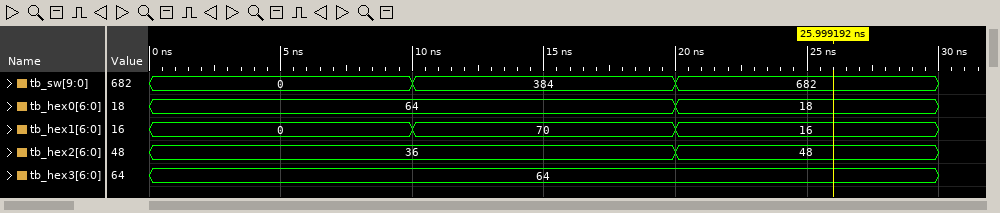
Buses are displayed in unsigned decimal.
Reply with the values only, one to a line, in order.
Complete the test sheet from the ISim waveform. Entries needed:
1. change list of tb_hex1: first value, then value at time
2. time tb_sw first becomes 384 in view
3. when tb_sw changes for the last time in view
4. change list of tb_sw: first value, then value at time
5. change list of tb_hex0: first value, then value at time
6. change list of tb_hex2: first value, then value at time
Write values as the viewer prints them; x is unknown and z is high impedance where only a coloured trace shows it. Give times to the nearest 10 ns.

0, 70 at 10 ns, 16 at 20 ns
10 ns
20 ns
0, 384 at 10 ns, 682 at 20 ns
64, 18 at 20 ns
36, 48 at 20 ns
